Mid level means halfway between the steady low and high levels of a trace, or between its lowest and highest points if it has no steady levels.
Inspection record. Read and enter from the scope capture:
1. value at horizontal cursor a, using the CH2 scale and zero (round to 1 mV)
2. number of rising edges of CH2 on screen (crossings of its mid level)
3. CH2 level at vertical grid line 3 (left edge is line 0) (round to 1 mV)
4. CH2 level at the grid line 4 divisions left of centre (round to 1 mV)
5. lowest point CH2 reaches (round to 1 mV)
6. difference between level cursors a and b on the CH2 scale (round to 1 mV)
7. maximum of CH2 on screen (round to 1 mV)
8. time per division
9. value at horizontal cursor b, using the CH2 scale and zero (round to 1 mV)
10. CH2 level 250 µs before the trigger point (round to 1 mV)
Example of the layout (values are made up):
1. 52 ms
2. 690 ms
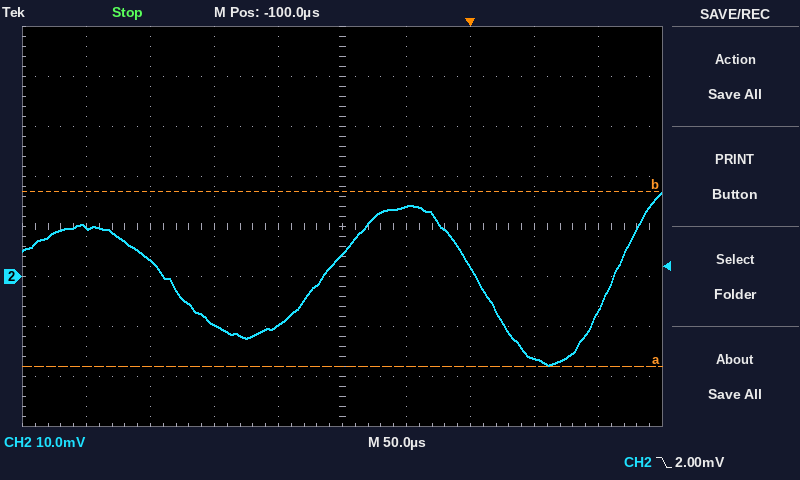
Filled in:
1. -18 mV
2. 2
3. -10 mV
4. 10 mV
5. -18 mV
6. 35 mV
7. 17 mV
8. 50 µs
9. 17 mV
10. 3 mV
